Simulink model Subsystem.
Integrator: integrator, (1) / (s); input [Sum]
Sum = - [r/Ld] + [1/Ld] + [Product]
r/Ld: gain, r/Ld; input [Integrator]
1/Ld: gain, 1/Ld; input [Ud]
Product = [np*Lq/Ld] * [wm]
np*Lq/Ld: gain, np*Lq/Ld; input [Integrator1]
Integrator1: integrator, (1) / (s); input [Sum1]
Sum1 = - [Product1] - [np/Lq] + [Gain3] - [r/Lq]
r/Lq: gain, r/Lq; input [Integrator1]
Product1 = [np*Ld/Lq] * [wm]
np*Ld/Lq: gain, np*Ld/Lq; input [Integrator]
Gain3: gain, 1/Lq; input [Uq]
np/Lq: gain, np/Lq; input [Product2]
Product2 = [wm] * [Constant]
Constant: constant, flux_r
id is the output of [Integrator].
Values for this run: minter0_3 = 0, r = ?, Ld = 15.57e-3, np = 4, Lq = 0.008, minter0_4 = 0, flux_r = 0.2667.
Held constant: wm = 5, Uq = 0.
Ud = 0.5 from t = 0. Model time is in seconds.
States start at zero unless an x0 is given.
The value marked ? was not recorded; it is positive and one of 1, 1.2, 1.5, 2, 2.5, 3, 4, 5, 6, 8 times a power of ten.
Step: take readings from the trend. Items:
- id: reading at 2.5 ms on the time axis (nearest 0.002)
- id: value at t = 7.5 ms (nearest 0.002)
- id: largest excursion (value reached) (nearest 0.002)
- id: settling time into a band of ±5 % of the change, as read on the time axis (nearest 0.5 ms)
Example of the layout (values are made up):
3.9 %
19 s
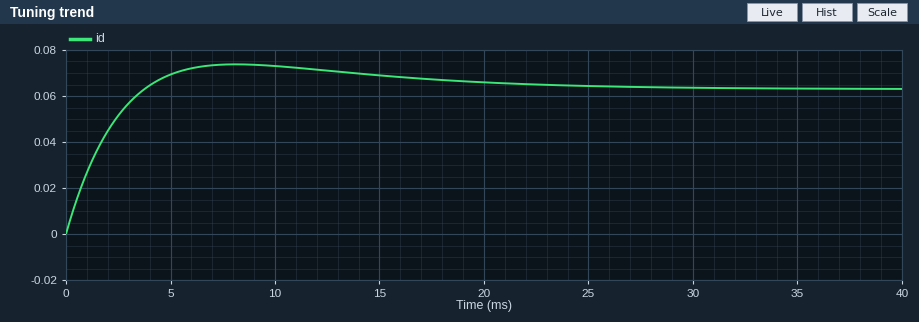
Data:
0.052
0.074
0.074
19.5 ms
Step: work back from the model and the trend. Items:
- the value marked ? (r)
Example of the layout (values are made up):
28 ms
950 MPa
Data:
2.5
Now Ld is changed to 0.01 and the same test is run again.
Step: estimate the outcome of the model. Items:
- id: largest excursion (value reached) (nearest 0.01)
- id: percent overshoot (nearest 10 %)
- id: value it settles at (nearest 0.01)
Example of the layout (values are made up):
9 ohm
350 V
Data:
0.09
40 %
0.06
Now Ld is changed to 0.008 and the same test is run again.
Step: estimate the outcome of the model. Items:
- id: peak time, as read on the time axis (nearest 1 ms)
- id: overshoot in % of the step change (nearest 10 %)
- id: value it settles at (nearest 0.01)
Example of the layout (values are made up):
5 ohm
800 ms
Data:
5 ms
50 %
0.06
